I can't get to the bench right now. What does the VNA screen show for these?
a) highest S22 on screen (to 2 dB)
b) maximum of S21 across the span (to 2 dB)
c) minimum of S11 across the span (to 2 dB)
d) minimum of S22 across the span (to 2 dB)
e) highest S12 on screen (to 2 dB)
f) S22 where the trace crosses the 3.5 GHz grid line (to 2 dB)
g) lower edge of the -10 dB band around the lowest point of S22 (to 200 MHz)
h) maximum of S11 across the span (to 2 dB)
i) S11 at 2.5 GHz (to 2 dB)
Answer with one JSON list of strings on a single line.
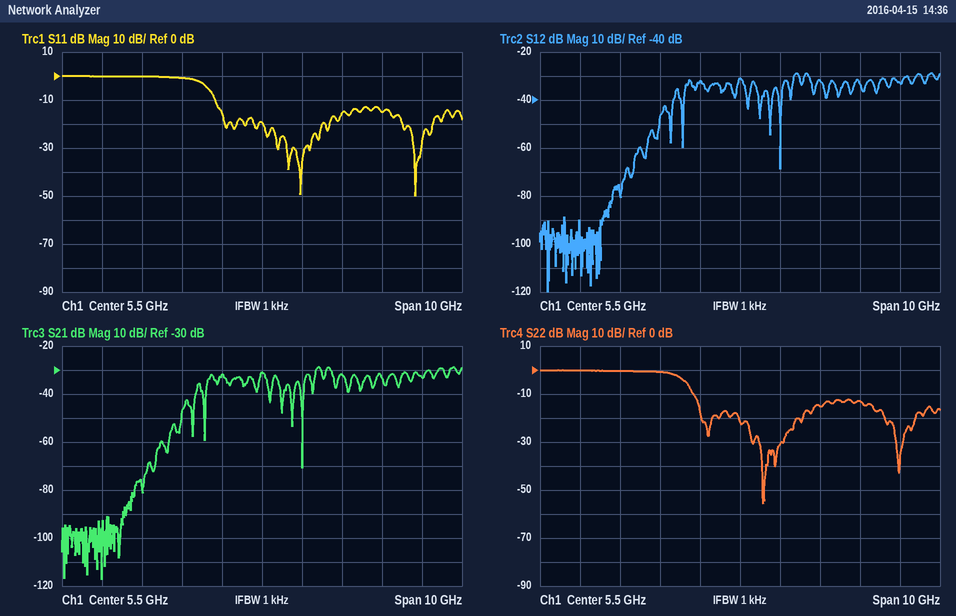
["0 dB", "-28 dB", "-50 dB", "-56 dB", "-28 dB", "0 dB", "4.4 GHz", "0 dB", "0 dB"]
